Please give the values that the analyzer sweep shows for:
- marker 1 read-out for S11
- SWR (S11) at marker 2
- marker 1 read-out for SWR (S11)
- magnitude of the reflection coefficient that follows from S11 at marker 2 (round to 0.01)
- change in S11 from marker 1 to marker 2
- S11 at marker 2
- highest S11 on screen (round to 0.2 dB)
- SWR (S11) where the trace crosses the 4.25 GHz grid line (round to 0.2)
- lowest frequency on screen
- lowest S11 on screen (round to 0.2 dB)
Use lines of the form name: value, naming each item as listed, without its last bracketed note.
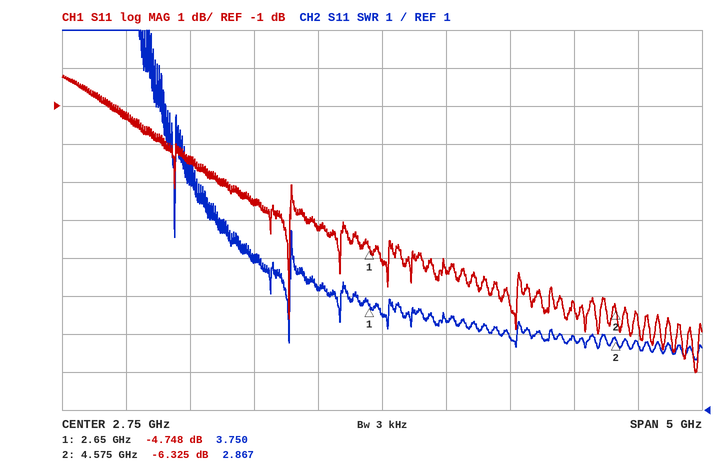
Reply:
marker 1 read-out for S11: -4.748 dB
SWR (S11) at marker 2: 2.867
marker 1 read-out for SWR: 3.750
magnitude of the reflection coefficient that follows from S11 at marker 2: 0.48
change in S11 from marker 1 to marker 2: -1.577 dB
S11 at marker 2: -6.325 dB
highest S11 on screen: -0.2 dB
SWR (S11) where the trace crosses the 4.25 GHz grid line: 3.0
lowest frequency on screen: 250 MHz
lowest S11 on screen: -8.0 dB
